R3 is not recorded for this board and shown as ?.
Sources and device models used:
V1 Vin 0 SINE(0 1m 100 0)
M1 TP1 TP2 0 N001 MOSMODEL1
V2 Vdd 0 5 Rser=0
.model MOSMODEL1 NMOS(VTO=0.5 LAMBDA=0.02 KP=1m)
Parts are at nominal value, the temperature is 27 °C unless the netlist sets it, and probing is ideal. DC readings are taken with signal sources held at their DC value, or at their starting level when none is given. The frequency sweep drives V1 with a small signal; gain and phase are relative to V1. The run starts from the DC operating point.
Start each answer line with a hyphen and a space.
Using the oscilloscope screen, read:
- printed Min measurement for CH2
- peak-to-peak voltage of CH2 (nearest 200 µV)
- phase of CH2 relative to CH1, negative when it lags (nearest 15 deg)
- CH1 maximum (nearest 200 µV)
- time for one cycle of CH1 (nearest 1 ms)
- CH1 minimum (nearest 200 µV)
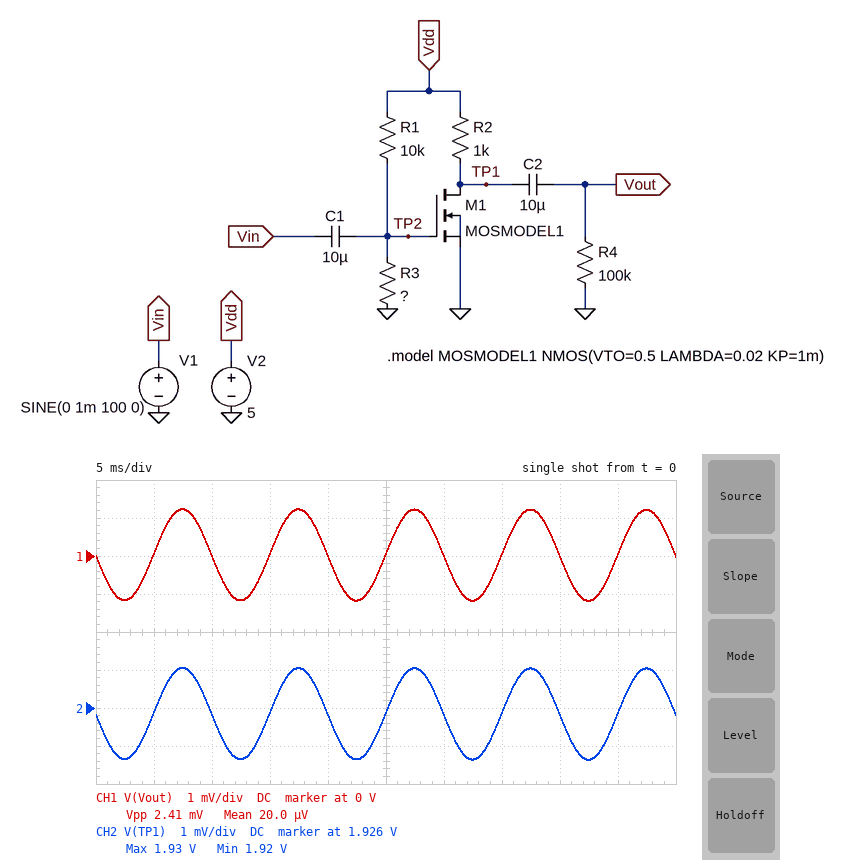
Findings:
- 1.92 V
- 2.4 mV
- 0 deg
- 1.2 mV
- 10 ms
- -1.2 mV
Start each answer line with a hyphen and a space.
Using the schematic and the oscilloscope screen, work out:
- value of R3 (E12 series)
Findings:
- 15 kΩ
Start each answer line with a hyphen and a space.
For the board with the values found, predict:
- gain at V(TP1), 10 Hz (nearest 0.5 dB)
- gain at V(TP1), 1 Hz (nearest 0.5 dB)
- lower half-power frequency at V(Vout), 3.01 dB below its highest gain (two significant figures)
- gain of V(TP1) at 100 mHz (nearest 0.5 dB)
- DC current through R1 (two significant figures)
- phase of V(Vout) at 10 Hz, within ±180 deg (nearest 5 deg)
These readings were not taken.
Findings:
- 1.5 dB
- -7.5 dB
- 2.7 Hz
- -27.0 dB
- 200 µA
- -165 deg
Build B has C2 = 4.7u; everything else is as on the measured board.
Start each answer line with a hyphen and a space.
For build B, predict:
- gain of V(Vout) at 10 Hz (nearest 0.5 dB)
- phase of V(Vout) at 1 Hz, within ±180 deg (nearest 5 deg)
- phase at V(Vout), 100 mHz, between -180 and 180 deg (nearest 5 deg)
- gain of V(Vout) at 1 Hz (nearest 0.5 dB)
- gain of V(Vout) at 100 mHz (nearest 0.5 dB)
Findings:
- 1.5 dB
- -90 deg
- -20 deg
- -8.0 dB
- -38.0 dB
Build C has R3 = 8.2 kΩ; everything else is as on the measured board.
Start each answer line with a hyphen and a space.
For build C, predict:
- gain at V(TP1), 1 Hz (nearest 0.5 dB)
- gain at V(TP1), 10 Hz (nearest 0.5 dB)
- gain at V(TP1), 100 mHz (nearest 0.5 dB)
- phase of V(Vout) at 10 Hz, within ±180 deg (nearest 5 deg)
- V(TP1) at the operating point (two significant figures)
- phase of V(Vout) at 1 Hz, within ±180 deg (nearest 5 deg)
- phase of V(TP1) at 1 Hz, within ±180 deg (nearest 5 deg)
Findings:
- -6.0 dB
- 4.5 dB
- -26.0 dB
- -160 deg
- 3.4 V
- -95 deg
- -105 deg
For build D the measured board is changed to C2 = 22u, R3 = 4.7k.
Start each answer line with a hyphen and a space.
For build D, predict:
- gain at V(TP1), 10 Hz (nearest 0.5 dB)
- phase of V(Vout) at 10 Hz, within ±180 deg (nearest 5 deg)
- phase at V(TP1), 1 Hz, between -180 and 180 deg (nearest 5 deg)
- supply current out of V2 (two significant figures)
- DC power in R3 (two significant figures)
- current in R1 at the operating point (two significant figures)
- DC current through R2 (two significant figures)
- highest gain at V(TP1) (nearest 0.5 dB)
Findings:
- 0.5 dB
- -155 deg
- -100 deg
- 1.0 mA
- 540 µW
- 340 µA
- 660 µA
- 1.5 dB
